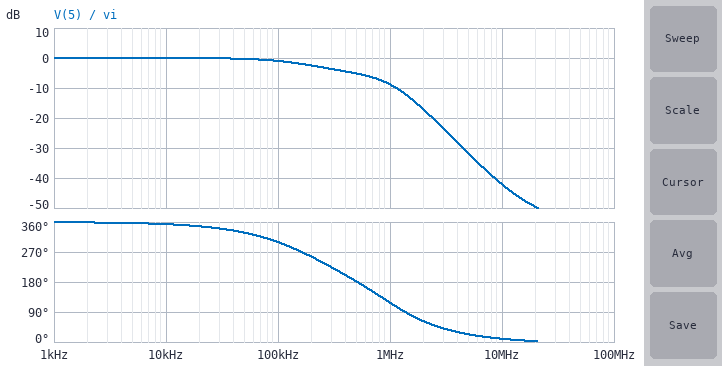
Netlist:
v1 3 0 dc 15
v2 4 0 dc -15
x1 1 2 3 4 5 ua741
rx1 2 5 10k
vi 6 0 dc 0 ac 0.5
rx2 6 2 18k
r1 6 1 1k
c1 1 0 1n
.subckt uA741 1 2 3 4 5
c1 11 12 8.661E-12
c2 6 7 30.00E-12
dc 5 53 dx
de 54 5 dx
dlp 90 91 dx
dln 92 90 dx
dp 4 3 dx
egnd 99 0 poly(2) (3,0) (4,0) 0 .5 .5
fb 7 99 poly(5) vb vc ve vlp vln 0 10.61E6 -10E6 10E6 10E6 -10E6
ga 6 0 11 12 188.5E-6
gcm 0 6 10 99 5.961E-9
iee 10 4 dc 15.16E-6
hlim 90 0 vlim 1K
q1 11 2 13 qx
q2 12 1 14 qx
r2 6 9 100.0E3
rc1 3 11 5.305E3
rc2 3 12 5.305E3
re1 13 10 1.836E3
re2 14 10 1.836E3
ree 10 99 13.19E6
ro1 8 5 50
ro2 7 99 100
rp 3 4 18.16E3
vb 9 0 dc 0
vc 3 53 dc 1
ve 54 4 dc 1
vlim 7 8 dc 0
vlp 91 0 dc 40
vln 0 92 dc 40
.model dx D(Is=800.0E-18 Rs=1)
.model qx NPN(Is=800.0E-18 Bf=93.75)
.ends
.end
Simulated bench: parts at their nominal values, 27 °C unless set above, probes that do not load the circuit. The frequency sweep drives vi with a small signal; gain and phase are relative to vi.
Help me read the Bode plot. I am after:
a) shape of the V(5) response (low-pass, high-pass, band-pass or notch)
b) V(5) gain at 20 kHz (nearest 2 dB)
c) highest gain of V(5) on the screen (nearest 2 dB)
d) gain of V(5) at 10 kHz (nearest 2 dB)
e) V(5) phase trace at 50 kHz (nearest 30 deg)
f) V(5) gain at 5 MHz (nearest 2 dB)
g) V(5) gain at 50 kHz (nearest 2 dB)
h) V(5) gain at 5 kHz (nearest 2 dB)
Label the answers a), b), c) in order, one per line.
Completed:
a) low-pass
b) 0 dB
c) 0 dB
d) 0 dB
e) 330 deg
f) -32 dB
g) 0 dB
h) 0 dB
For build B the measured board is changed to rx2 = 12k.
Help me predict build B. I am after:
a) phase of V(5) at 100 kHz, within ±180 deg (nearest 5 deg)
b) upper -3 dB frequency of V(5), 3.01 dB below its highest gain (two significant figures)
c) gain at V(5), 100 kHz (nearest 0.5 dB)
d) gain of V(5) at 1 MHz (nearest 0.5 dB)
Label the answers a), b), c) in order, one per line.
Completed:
a) -70 deg
b) 520 kHz
c) -0.5 dB
d) -7.0 dB
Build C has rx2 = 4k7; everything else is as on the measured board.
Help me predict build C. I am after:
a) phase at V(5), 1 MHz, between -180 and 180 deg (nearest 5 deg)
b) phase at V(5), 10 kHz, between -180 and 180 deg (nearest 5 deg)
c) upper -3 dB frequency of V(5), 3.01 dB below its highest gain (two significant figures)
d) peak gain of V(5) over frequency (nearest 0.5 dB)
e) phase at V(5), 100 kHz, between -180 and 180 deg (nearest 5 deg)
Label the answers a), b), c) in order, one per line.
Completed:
a) 90 deg
b) -15 deg
c) 570 kHz
d) 4.0 dB
e) -105 deg
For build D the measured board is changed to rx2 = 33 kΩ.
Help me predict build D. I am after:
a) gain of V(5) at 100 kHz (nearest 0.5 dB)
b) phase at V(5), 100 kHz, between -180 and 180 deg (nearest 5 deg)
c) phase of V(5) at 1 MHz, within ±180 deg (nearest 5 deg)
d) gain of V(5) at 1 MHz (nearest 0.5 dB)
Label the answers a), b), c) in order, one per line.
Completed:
a) -1.5 dB
b) -50 deg
c) 135 deg
d) -12.0 dB
